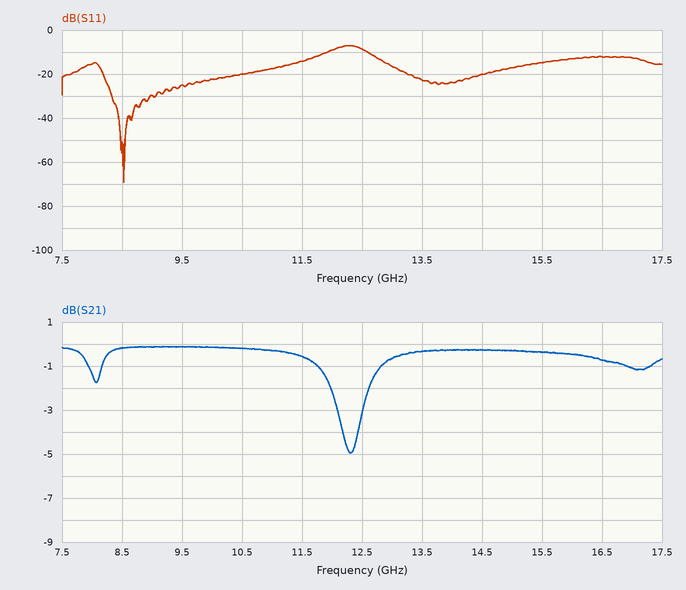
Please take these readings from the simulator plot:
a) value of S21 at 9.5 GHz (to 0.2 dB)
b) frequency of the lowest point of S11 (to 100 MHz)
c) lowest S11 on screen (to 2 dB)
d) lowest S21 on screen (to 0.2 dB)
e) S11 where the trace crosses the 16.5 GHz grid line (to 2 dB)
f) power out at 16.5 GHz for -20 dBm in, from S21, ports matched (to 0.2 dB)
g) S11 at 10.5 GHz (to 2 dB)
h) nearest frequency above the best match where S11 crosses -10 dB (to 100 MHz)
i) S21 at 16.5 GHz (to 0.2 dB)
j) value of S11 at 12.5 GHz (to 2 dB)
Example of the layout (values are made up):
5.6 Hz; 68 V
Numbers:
-0.2 dB; 8.5 GHz; -70 dB; -5.0 dB; -12 dB; -20.8 dBm; -20 dB; 11.9 GHz; -0.8 dB; -8 dB
